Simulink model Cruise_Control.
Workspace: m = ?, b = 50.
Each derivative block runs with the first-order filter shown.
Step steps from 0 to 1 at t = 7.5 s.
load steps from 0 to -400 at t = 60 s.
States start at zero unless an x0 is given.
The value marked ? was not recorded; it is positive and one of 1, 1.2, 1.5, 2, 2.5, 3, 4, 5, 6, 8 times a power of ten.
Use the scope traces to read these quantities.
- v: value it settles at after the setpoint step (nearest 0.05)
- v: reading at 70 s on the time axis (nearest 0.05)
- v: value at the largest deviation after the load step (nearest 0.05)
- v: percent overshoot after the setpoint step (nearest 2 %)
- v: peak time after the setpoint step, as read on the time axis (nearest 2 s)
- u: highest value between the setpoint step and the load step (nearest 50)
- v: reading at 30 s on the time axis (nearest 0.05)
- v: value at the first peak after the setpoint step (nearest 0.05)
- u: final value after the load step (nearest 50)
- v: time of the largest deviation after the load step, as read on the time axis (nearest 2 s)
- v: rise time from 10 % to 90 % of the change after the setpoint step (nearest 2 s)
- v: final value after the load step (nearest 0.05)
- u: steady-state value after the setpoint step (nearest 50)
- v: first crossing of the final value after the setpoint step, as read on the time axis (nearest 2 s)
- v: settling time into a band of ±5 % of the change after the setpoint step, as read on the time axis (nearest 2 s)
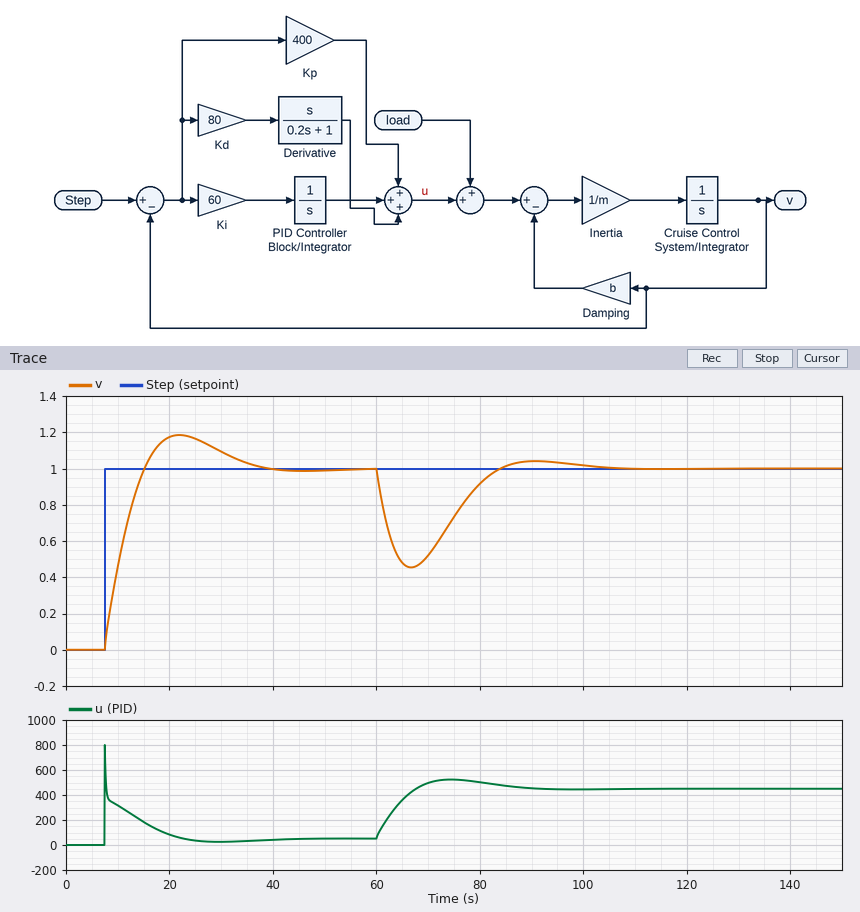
1.00
0.50
0.45
18 %
22 s
800
1.10
1.20
450
66 s
6 s
1.00
50
16 s
34 s
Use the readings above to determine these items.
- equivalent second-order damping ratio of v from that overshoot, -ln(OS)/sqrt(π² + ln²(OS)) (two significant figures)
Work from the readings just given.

0.48
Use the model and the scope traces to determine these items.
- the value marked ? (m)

2000
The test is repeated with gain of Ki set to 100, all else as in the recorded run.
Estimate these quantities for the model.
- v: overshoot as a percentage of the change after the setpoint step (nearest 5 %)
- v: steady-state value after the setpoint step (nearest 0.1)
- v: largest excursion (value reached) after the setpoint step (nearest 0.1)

25 %
1.0
1.3
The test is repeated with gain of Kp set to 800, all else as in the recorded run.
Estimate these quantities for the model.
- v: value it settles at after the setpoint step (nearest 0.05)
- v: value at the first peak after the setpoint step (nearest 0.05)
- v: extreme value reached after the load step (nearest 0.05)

1.00
1.05
0.65
